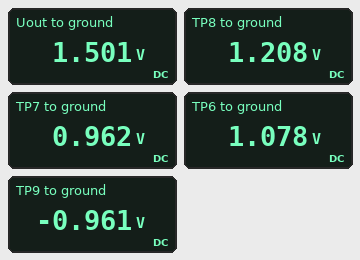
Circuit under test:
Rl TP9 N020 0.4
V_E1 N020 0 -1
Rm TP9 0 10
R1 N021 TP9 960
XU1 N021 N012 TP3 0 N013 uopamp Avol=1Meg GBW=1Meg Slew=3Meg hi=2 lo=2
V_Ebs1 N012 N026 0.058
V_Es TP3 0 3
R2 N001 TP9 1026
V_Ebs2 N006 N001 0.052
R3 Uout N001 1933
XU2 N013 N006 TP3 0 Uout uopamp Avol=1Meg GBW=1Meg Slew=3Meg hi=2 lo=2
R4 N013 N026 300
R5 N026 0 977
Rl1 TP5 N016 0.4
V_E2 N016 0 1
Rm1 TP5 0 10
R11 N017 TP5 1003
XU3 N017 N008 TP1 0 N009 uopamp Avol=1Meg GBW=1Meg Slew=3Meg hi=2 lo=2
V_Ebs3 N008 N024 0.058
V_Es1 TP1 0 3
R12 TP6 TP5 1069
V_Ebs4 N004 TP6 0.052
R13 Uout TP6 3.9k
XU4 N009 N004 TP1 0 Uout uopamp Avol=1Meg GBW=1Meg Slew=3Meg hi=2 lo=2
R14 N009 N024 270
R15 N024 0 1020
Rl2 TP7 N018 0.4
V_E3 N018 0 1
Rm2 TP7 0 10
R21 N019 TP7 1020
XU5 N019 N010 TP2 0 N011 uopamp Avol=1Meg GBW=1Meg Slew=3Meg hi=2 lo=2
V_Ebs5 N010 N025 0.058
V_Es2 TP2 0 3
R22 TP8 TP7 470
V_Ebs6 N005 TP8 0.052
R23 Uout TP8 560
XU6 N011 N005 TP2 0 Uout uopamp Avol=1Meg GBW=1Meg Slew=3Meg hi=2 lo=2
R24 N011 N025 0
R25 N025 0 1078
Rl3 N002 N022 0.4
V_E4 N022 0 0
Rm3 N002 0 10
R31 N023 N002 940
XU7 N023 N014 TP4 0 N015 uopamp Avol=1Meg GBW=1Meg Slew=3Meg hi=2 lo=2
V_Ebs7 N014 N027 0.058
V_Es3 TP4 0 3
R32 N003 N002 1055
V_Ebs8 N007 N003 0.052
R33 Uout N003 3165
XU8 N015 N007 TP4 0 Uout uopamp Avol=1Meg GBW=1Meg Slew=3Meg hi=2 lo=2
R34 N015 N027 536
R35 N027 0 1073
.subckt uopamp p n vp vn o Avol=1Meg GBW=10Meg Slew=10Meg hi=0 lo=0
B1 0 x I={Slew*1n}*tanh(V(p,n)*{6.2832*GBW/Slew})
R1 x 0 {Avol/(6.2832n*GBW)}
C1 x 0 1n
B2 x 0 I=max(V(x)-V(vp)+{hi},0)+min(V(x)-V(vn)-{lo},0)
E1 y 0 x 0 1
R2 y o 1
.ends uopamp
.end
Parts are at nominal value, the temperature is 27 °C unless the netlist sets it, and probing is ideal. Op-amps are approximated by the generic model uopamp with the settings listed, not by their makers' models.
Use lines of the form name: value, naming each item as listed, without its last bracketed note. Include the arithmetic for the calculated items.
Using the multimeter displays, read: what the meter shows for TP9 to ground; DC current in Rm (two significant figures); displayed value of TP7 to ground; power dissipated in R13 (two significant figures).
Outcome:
what the meter shows for TP9 to ground: -0.961 V
DC current in Rm: (0 V - (-961 mV)) / 10 Ω = 96 mA
displayed value of TP7 to ground: 0.962 V
power dissipated in R13: (1.501 V - 1.078 V)^2 / 3.9 kΩ = 46 µW
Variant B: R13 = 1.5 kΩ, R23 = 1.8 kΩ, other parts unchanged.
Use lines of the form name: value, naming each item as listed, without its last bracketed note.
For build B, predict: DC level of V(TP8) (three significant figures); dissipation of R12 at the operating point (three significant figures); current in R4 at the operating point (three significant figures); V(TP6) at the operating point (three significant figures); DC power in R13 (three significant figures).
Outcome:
DC level of V(TP8): 1.07 V
dissipation of R12 at the operating point: 47.1 µW
current in R4 at the operating point: 1.17 mA
V(TP6) at the operating point: 1.19 V
DC power in R13: 66.1 µW
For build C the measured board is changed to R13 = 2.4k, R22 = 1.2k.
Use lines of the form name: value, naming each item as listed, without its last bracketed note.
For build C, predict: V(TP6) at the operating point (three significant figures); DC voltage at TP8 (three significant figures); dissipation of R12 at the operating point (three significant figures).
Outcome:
V(TP6) at the operating point: 1.13 V
DC voltage at TP8: 1.33 V
dissipation of R12 at the operating point: 25.8 µW
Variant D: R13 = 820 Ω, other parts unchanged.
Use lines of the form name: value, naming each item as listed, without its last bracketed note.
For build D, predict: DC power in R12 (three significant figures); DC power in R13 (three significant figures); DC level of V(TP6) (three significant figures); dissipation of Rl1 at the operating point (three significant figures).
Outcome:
DC power in R12: 87.0 µW
DC power in R13: 66.7 µW
DC level of V(TP6): 1.27 V
dissipation of Rl1 at the operating point: 3.68 mW
